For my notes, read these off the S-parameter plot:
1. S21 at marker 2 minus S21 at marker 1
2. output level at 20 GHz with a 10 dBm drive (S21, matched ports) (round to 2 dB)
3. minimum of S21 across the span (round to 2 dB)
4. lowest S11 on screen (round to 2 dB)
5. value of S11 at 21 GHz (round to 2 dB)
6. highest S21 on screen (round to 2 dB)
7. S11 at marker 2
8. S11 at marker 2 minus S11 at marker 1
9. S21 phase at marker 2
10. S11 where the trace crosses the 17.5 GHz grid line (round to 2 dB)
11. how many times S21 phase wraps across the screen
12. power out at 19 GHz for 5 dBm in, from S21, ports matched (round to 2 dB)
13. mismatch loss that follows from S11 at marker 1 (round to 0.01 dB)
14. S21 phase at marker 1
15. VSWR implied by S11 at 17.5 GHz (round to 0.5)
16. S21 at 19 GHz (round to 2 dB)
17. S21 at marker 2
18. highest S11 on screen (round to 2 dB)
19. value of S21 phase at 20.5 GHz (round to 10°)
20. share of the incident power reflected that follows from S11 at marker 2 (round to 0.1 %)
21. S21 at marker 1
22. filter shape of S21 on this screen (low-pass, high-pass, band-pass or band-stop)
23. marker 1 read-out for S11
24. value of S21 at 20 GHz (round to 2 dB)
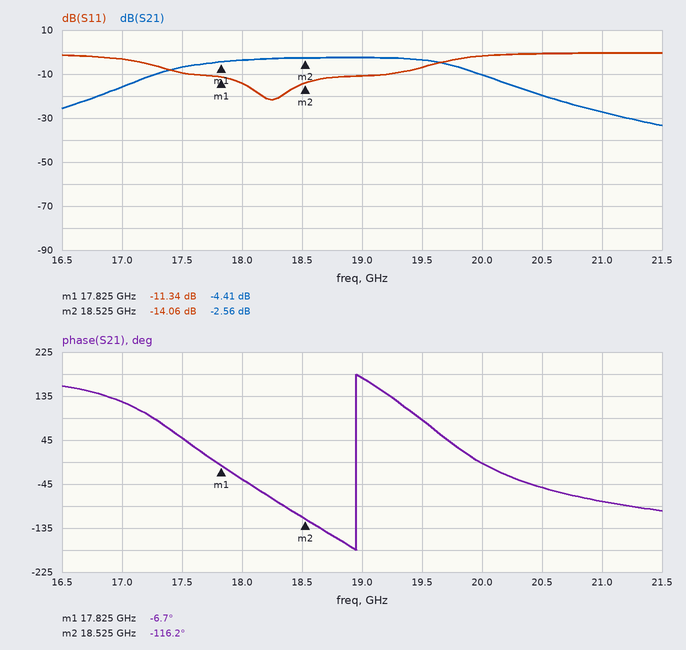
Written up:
1.85 dB
0 dBm
-34 dB
-22 dB
0 dB
-2 dB
-14.06 dB
-2.72 dB
-116.2°
-10 dB
1
2 dBm
0.33 dB
-6.7°
2.0
-2 dB
-2.56 dB
0 dB
-50°
3.9 %
-4.41 dB
band-pass
-11.34 dB
-10 dB
